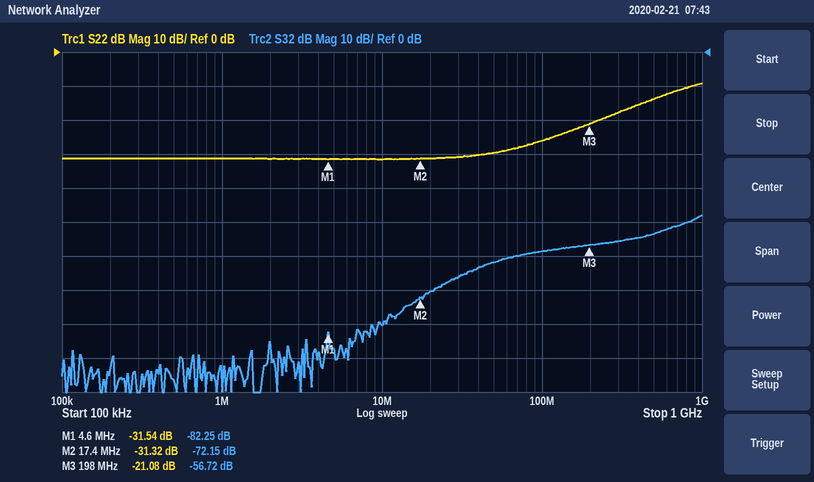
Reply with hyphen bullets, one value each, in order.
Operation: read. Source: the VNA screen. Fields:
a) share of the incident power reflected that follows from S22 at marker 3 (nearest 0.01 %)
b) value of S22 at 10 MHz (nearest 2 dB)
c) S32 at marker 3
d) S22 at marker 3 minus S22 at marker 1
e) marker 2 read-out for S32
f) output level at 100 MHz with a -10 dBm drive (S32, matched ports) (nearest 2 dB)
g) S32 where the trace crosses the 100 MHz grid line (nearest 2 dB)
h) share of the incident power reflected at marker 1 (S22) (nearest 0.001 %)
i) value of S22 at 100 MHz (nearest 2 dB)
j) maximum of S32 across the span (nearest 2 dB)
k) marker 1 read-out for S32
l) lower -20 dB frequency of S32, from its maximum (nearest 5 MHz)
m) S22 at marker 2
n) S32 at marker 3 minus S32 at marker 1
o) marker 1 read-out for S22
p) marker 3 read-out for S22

- 0.78 %
- -32 dB
- -56.72 dB
- 10.46 dB
- -72.15 dB
- -68 dBm
- -58 dB
- 0.070 %
- -26 dB
- -48 dB
- -82.25 dB
- 25 MHz
- -31.32 dB
- 25.53 dB
- -31.54 dB
- -21.08 dB
